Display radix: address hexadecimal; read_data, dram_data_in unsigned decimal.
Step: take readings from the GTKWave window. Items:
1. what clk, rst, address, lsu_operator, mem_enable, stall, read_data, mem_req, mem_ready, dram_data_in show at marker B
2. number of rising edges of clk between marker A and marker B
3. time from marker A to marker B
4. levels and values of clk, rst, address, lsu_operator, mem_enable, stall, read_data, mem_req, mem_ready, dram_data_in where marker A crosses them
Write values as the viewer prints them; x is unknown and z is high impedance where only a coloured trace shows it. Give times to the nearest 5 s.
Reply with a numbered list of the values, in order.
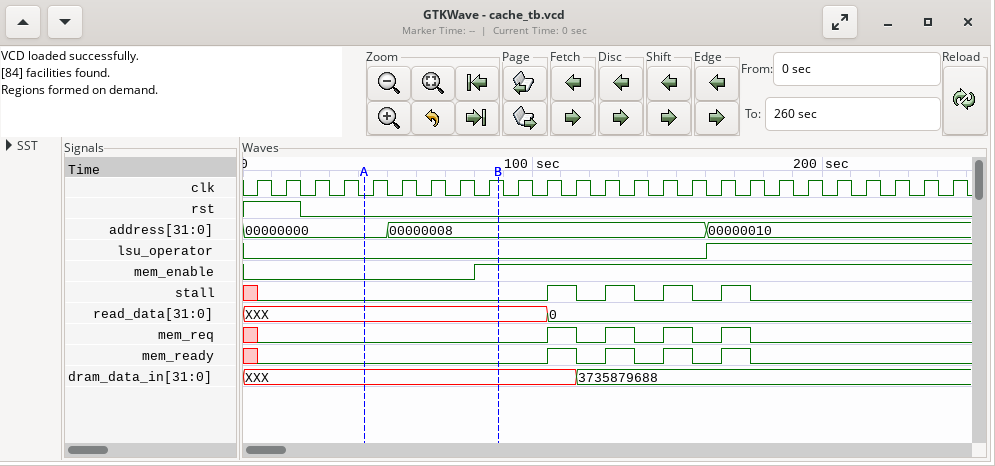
1. clk=1, rst=0, address=00000008, lsu_operator=0, mem_enable=1, stall=0, read_data=XXX, mem_req=0, mem_ready=0, dram_data_in=XXX
2. 5
3. 45 s
4. clk=0, rst=0, address=00000000, lsu_operator=0, mem_enable=0, stall=0, read_data=XXX, mem_req=0, mem_ready=0, dram_data_in=XXX
